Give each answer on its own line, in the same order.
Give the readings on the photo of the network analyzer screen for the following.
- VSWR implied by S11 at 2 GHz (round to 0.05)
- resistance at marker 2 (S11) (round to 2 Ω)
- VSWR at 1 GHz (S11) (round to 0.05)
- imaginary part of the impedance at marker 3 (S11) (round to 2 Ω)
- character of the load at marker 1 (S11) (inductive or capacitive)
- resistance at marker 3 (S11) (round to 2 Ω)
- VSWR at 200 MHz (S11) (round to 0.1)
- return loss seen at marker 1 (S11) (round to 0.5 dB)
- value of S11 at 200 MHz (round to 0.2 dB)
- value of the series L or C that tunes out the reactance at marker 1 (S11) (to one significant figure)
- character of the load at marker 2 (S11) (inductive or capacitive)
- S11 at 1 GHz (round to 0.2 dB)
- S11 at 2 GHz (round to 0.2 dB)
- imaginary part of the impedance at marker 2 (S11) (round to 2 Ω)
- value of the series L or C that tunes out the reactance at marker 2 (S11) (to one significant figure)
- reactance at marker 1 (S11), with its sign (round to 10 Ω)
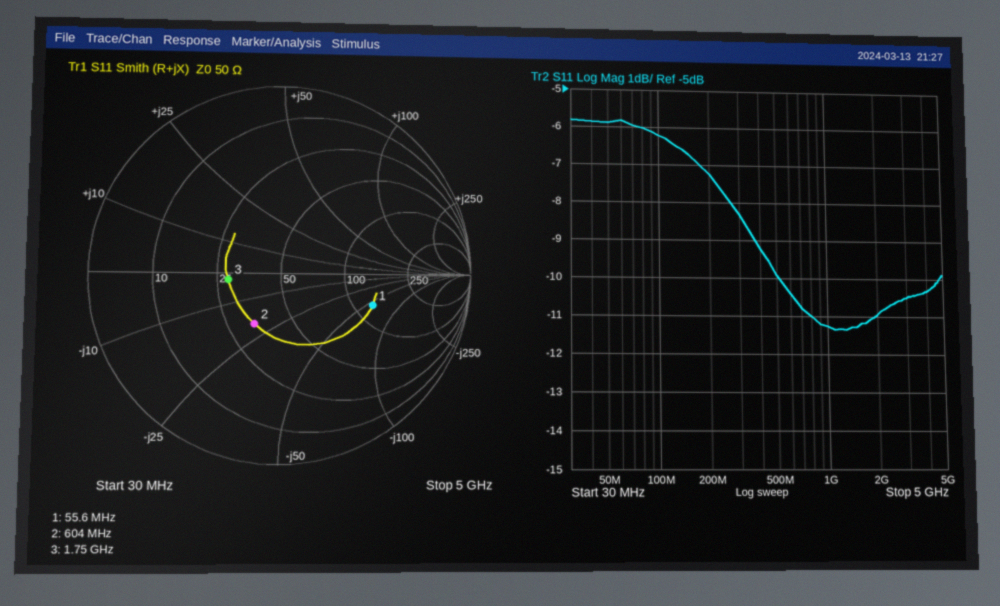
1.80
34 Ω
1.75
-2 Ω
capacitive
28 Ω
2.5
6.0 dB
-7.2 dB
200 nH
capacitive
-11.2 dB
-11.0 dB
-20 Ω
5 nH
-60 Ω
